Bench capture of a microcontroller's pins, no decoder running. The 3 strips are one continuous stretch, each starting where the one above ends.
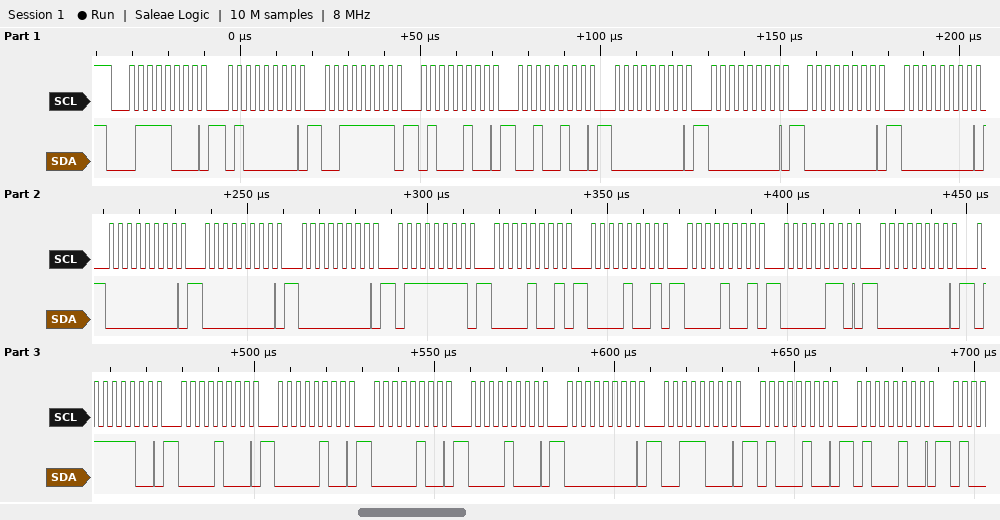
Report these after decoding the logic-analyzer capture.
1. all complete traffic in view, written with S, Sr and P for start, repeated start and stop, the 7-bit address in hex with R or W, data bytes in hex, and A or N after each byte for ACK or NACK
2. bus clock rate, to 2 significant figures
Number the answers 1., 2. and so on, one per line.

1. S 3CW A 40 A 3F A 44 A 24 A 00 A 00 A 00 A 00 A 00 A 00 A 00 A 7F A 09 A 09 A 09 A 06 A 00 A 7C A 08 A 04 A 04 A 08 A 00 A 38 A 44 A 44 A
2. 400 kHz
